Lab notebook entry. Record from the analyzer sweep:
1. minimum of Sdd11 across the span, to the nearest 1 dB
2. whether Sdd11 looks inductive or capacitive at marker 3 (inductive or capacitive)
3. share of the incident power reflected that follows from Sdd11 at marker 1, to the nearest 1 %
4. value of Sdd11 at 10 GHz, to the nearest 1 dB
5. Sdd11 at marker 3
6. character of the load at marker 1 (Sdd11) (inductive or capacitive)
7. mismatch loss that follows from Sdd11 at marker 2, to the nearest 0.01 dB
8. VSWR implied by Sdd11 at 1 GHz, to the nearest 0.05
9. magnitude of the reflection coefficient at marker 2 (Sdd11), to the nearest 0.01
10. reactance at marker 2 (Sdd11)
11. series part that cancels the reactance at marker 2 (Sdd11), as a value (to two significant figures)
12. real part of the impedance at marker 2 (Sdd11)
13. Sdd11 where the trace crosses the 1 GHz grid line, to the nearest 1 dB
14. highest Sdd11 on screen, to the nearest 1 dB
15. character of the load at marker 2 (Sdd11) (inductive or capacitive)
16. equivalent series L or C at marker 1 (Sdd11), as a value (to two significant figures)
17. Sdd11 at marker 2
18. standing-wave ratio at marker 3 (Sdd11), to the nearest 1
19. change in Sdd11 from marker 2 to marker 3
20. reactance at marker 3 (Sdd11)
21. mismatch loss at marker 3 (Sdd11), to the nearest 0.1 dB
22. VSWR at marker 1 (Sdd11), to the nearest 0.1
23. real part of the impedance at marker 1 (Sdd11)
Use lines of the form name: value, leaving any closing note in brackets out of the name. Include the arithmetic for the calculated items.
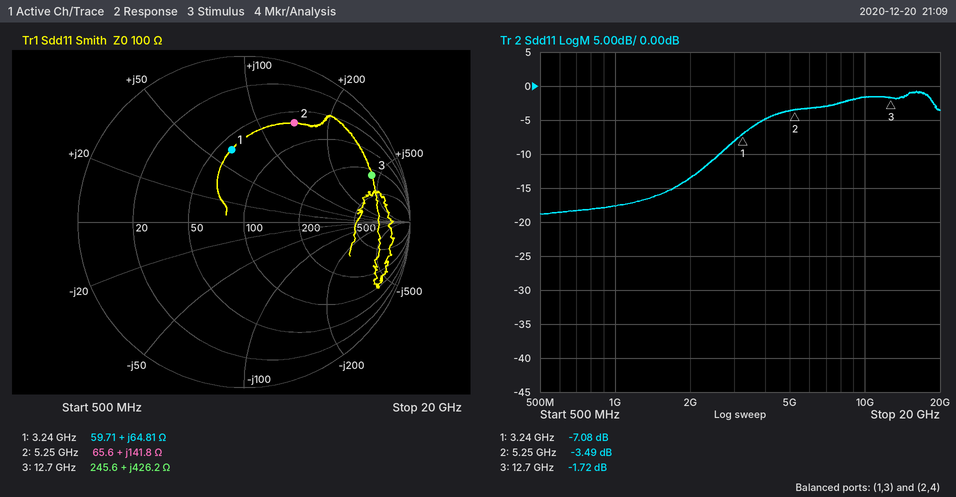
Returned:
minimum of Sdd11 across the span, to the nearest 1 dB: -19 dB
whether Sdd11 looks inductive or capacitive at marker 3: inductive
share of the incident power reflected that follows from Sdd11 at marker 1, to the nearest 1 %: 10^(-7.08/10) ≈ 20 %
value of Sdd11 at 10 GHz, to the nearest 1 dB: -2 dB
Sdd11 at marker 3: -1.72 dB
character of the load at marker 1 (Sdd11): inductive
mismatch loss that follows from Sdd11 at marker 2, to the nearest 0.01 dB: −10 log10(1 − 10^(-3.49/10)) ≈ 2.58 dB
VSWR implied by Sdd11 at 1 GHz, to the nearest 0.05: |Γ| = 10^(-18/20) = 0.1259; VSWR = (1 + 0.1259)/(1 − 0.1259) ≈ 1.29, so 1.30 to the nearest 0.05
magnitude of the reflection coefficient at marker 2 (Sdd11), to the nearest 0.01: 0.67
reactance at marker 2: +141.8 Ω
series part that cancels the reactance at marker 2 (Sdd11), as a value: C = 1/(2π × 5.25 GHz × 141.8 Ω) ≈ 214 fF, so 210 fF to two significant figures
real part of the impedance at marker 2: 65.6 Ω
Sdd11 where the trace crosses the 1 GHz grid line, to the nearest 1 dB: -18 dB
highest Sdd11 on screen, to the nearest 1 dB: -1 dB
character of the load at marker 2 (Sdd11): inductive
equivalent series L or C at marker 1 (Sdd11), as a value: L = 64.81 Ω/(2π × 3.24 GHz) ≈ 3.2 nH
Sdd11 at marker 2: -3.49 dB
standing-wave ratio at marker 3 (Sdd11), to the nearest 1: 10
change in Sdd11 from marker 2 to marker 3: -1.72 − (-3.49) = 1.77 dB
reactance at marker 3: +426.2 Ω
mismatch loss at marker 3 (Sdd11), to the nearest 0.1 dB: −10 log10(1 − 10^(-1.72/10)) ≈ 4.9 dB
VSWR at marker 1 (Sdd11), to the nearest 0.1: 2.6
real part of the impedance at marker 1: 59.71 Ω
